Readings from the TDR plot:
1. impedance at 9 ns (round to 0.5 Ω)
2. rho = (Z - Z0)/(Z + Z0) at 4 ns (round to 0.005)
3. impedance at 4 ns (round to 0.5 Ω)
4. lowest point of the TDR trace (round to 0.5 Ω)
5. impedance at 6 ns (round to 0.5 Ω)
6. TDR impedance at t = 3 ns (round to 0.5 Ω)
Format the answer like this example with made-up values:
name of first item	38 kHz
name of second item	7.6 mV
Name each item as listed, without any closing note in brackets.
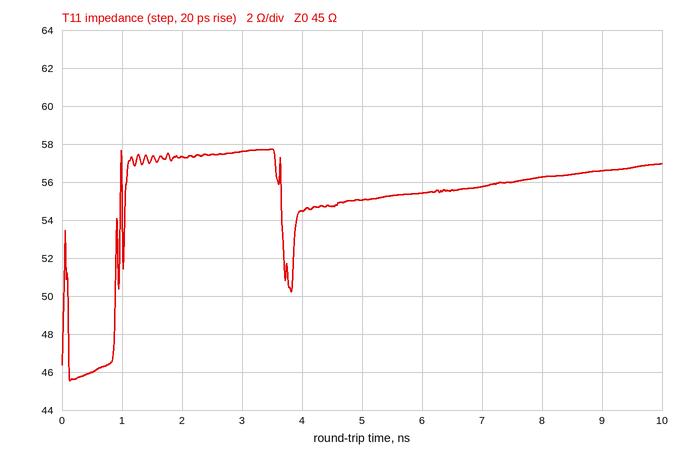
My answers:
impedance at 9 ns	56.5 Ω
rho = (Z - Z0)/(Z + Z0) at 4 ns	+0.095
impedance at 4 ns	54.5 Ω
lowest point of the TDR trace	45.5 Ω
impedance at 6 ns	55.5 Ω
TDR impedance at t = 3 ns	57.5 Ω
